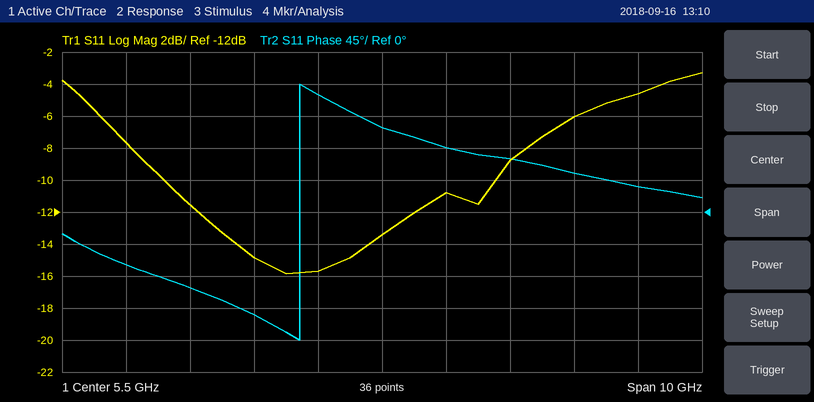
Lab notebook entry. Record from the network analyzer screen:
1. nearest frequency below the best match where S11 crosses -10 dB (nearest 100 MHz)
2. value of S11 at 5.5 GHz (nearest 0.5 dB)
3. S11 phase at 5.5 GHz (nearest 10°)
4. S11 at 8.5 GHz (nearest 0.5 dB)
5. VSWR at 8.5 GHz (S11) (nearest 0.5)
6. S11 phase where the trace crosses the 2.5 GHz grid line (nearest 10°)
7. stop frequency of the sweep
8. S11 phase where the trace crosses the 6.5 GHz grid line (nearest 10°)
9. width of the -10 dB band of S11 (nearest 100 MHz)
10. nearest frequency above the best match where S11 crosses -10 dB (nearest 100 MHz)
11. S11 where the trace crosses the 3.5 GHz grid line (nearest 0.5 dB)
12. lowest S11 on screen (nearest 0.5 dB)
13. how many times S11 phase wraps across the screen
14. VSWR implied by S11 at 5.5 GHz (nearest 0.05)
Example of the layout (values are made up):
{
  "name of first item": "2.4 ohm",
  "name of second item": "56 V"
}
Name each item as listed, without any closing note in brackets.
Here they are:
{
  "nearest frequency below the best match where S11 crosses -10 dB": "2.1 GHz",
  "value of S11 at 5.5 GHz": "-13.5 dB",
  "S11 phase at 5.5 GHz": "120°",
  "S11 at 8.5 GHz": "-6.0 dB",
  "VSWR at 8.5 GHz (S11)": "3.0",
  "S11 phase where the trace crosses the 2.5 GHz grid line": "-110°",
  "stop frequency of the sweep": "10.5 GHz",
  "S11 phase where the trace crosses the 6.5 GHz grid line": "90°",
  "width of the -10 dB band of S11": "5.2 GHz",
  "nearest frequency above the best match where S11 crosses -10 dB": "7.3 GHz",
  "S11 where the trace crosses the 3.5 GHz grid line": "-15.0 dB",
  "lowest S11 on screen": "-16.0 dB",
  "how many times S11 phase wraps across the screen": "1",
  "VSWR implied by S11 at 5.5 GHz": "1.55"
}
